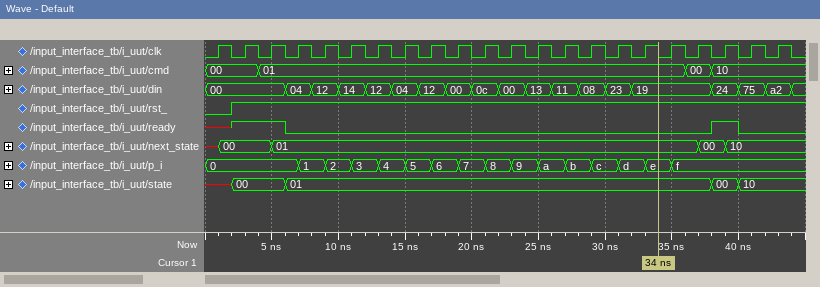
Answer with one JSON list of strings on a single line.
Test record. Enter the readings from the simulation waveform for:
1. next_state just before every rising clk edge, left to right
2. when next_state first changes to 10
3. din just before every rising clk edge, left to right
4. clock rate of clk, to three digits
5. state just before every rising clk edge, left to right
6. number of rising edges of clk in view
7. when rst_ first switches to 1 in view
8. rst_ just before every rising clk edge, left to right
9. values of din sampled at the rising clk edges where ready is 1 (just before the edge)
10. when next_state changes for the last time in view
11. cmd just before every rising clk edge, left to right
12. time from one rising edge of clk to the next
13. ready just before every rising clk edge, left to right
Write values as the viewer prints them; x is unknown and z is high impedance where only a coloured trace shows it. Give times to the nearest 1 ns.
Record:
["x, 00, 00, 01, 01, 01, 01, 01, 01, 01, 01, 01, 01, 01, 01, 01, 01, 01, 01, 00, 10, 10", "39 ns", "00, 00, 00, 04, 12, 14, 12, 04, 12, 00, 0c, 00, 13, 11, 08, 23, 19, 19, 19, 24, 75, a2", "500 MHz", "x, 00, 00, 01, 01, 01, 01, 01, 01, 01, 01, 01, 01, 01, 01, 01, 01, 01, 01, 00, 10, 10", "22", "2 ns", "0 1 1 1 1 1 1 1 1 1 1 1 1 1 1 1 1 1 1 1 1 1", "00, 00, 24", "39 ns", "00, 00, 01, 01, 01, 01, 01, 01, 01, 01, 01, 01, 01, 01, 01, 01, 01, 01, 00, 10, 10, 10", "2 ns", "x 1 1 0 0 0 0 0 0 0 0 0 0 0 0 0 0 0 0 1 0 0"]
